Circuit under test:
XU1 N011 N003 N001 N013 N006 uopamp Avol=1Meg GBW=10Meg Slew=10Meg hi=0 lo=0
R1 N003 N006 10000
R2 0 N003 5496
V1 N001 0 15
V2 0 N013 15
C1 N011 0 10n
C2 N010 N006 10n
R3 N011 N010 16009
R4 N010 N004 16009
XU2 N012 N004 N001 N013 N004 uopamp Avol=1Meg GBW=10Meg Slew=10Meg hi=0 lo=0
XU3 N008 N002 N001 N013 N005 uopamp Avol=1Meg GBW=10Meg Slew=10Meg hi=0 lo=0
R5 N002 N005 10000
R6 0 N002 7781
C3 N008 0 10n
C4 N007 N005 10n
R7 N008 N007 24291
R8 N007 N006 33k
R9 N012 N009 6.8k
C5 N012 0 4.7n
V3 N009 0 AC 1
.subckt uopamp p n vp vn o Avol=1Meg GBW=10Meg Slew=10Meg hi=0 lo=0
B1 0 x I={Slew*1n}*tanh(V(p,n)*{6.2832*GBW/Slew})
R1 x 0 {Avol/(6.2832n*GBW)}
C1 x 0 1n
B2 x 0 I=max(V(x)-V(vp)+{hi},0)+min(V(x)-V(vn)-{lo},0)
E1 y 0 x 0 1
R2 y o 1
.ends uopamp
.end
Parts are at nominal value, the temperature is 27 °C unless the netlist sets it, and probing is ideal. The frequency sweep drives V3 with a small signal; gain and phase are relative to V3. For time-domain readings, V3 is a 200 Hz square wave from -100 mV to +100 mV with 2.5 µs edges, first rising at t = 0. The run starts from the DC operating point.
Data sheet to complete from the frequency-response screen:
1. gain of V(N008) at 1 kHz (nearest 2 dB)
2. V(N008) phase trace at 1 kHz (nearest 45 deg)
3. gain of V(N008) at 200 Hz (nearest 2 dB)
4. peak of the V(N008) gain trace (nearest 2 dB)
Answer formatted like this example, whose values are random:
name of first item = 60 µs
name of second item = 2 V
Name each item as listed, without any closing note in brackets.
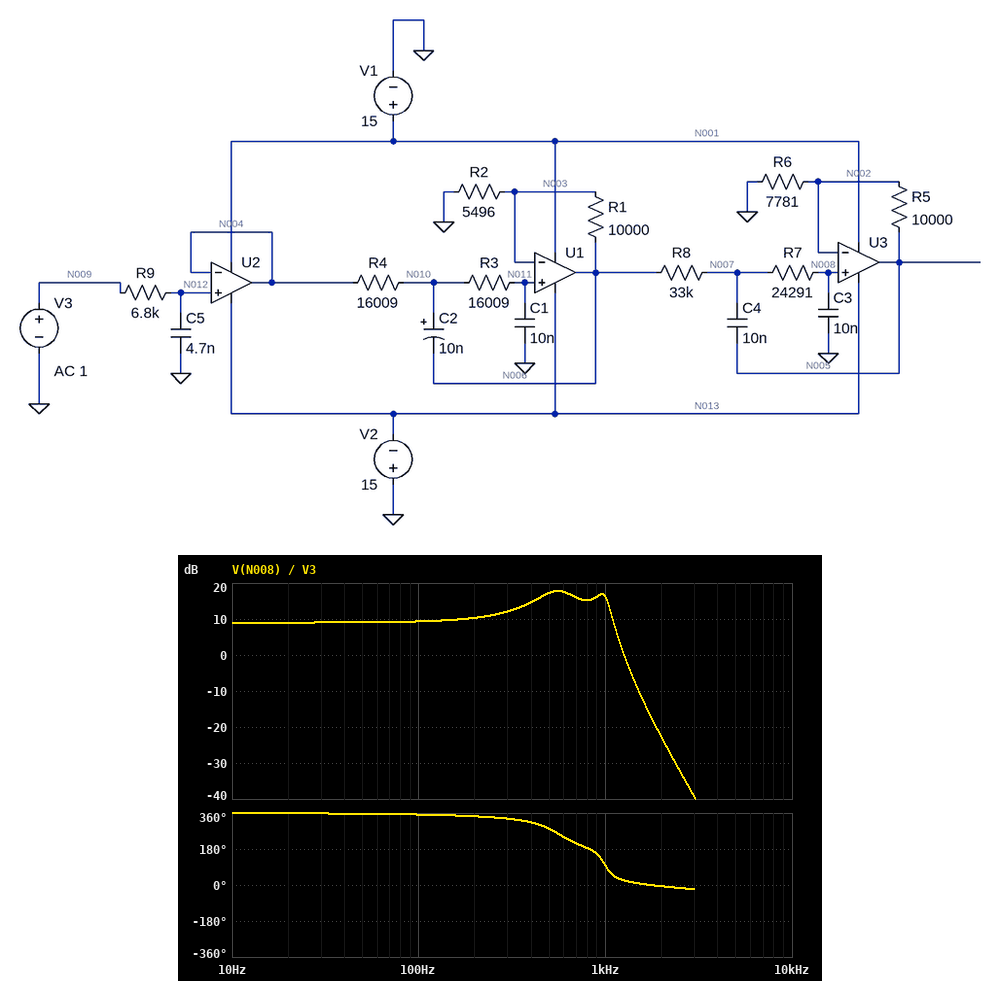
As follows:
gain of V(N008) at 1 kHz = 16 dB
V(N008) phase trace at 1 kHz = 90 deg
gain of V(N008) at 200 Hz = 10 dB
peak of the V(N008) gain trace = 18 dB
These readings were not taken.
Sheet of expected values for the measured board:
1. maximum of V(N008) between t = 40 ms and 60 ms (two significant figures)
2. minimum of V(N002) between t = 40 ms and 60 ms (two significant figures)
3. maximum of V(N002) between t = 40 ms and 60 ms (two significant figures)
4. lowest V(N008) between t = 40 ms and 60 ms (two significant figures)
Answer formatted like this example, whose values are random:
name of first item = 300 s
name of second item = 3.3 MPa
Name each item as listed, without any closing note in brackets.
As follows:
maximum of V(N008) between t = 40 ms and 60 ms = 830 mV
minimum of V(N002) between t = 40 ms and 60 ms = -830 mV
maximum of V(N002) between t = 40 ms and 60 ms = 830 mV
lowest V(N008) between t = 40 ms and 60 ms = -830 mV
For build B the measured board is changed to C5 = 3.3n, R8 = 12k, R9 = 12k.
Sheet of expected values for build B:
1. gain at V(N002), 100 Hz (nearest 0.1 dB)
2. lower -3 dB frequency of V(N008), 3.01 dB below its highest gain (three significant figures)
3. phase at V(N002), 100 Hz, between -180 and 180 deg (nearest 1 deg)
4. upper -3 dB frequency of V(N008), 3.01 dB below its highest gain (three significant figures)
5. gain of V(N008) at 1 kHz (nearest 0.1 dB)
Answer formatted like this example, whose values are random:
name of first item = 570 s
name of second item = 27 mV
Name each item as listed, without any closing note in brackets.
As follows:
gain at V(N002), 100 Hz = 9.1 dB
lower -3 dB frequency of V(N008), 3.01 dB below its highest gain = 865 Hz
phase at V(N002), 100 Hz, between -180 and 180 deg = -10 deg
upper -3 dB frequency of V(N008), 3.01 dB below its highest gain = 1.06 kHz
gain of V(N008) at 1 kHz = 21.1 dB
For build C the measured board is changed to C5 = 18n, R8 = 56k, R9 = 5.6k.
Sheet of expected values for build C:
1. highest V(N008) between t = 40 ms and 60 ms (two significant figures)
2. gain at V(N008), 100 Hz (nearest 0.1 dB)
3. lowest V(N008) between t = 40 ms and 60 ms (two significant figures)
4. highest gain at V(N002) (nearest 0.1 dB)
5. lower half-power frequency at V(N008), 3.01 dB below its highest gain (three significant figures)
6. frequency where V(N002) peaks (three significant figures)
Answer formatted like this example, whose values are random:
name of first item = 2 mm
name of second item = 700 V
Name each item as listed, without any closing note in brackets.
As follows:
highest V(N008) between t = 40 ms and 60 ms = 660 mV
gain at V(N008), 100 Hz = 9.5 dB
lowest V(N008) between t = 40 ms and 60 ms = -660 mV
highest gain at V(N002) = 23.4 dB
lower half-power frequency at V(N008), 3.01 dB below its highest gain = 378 Hz
frequency where V(N002) peaks = 428 Hz
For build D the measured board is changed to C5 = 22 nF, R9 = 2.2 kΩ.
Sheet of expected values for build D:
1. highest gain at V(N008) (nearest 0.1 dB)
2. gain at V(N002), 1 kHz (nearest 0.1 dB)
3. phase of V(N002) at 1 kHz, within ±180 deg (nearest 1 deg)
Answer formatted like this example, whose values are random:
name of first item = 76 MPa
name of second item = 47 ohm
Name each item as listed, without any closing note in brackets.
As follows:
highest gain at V(N008) = 17.7 dB
gain at V(N002), 1 kHz = 16.0 dB
phase of V(N002) at 1 kHz, within ±180 deg = 92 deg
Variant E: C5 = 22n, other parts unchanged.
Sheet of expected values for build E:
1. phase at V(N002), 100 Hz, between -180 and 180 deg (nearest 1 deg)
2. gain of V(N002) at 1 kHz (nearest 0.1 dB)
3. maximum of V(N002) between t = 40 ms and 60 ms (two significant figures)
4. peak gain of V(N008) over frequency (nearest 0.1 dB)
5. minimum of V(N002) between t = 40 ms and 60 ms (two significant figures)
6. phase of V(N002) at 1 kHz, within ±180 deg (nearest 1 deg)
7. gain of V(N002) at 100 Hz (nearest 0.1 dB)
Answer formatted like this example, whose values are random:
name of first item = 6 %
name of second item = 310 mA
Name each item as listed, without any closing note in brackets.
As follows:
phase at V(N002), 100 Hz, between -180 and 180 deg = -12 deg
gain of V(N002) at 1 kHz = 13.6 dB
maximum of V(N002) between t = 40 ms and 60 ms = 730 mV
peak gain of V(N008) over frequency = 16.8 dB
minimum of V(N002) between t = 40 ms and 60 ms = -730 mV
phase of V(N002) at 1 kHz, within ±180 deg = 66 deg
gain of V(N002) at 100 Hz = 9.3 dB
